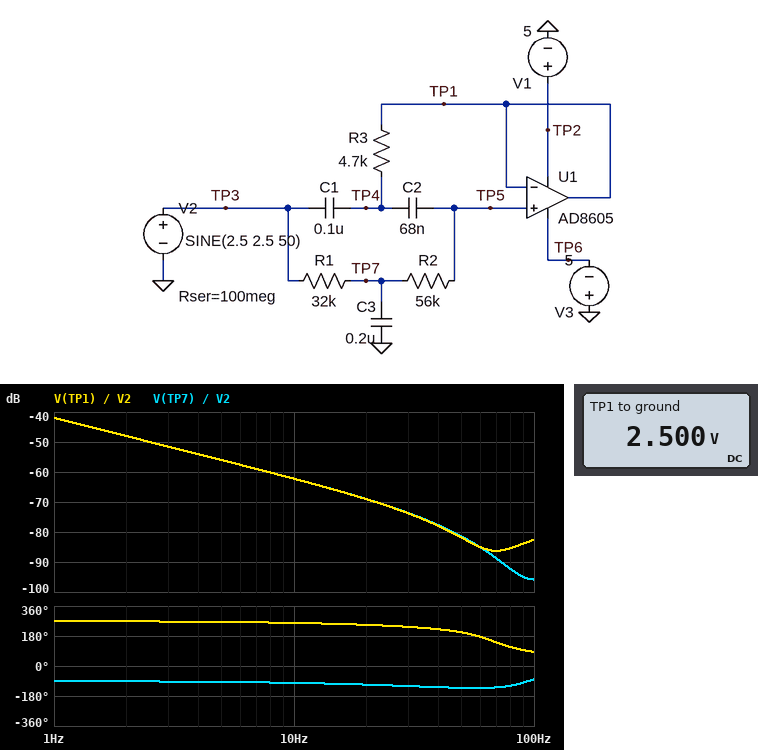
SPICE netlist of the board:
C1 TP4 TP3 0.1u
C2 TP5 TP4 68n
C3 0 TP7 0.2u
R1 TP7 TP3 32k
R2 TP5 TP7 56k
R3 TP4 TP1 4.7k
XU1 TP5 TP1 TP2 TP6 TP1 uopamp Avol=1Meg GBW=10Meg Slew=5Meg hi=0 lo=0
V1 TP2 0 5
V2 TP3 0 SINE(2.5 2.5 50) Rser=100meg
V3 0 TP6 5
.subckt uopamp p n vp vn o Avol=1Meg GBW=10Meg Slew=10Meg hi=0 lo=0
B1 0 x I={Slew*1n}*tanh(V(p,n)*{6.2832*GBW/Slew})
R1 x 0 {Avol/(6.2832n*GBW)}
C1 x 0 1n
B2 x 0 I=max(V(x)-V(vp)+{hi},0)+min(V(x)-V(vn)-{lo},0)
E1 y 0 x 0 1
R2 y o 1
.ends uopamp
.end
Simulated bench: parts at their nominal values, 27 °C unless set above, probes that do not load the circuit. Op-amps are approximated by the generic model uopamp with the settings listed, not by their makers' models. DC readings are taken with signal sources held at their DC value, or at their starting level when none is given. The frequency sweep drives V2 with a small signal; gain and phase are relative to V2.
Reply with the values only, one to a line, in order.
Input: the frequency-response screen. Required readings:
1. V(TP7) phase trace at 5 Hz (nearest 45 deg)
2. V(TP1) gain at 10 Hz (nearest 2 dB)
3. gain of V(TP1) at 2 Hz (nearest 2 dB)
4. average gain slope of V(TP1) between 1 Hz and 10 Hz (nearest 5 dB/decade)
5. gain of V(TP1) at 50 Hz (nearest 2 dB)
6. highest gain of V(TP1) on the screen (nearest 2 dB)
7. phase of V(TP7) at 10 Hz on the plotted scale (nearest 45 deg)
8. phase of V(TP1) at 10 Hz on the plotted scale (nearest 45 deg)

-90 deg
-62 dB
-48 dB
-20 dB/decade
-82 dB
-42 dB
-90 deg
270 deg
